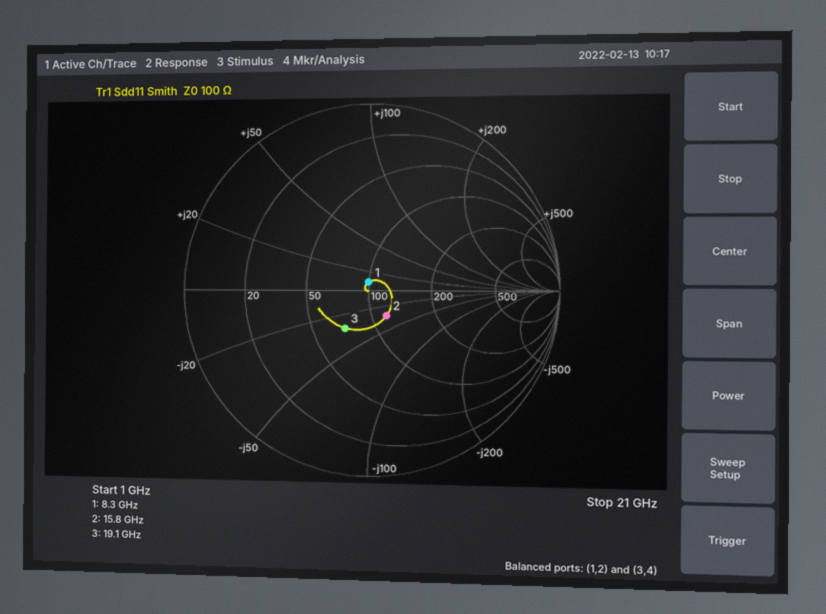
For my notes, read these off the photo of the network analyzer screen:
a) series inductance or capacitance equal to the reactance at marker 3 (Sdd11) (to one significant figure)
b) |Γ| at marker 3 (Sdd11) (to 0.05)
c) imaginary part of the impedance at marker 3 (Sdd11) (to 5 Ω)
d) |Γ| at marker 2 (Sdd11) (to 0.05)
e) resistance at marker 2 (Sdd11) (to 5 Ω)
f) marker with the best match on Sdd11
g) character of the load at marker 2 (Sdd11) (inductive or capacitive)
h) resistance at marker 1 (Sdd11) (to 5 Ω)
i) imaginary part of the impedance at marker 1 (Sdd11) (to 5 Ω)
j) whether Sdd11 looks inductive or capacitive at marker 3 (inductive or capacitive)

300 fF
0.25
-30 Ω
0.15
115 Ω
marker 1
capacitive
100 Ω
+10 Ω
capacitive
